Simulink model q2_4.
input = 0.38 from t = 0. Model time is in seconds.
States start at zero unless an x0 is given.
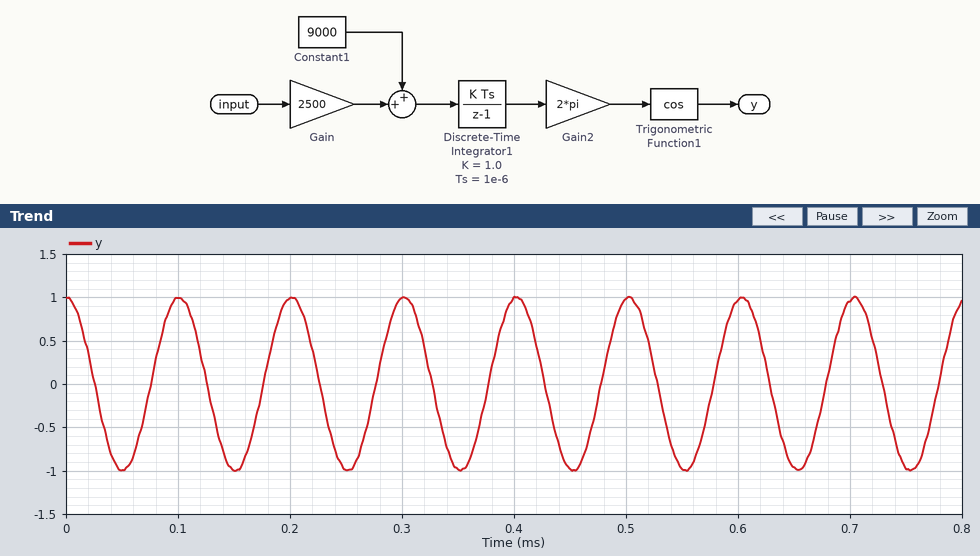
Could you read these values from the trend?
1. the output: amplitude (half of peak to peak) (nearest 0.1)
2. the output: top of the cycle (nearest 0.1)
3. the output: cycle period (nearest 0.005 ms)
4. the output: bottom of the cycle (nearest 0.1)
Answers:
1.0
1.0
0.100 ms
-1.0
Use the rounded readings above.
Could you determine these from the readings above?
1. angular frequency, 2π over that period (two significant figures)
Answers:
63 rad/ms
